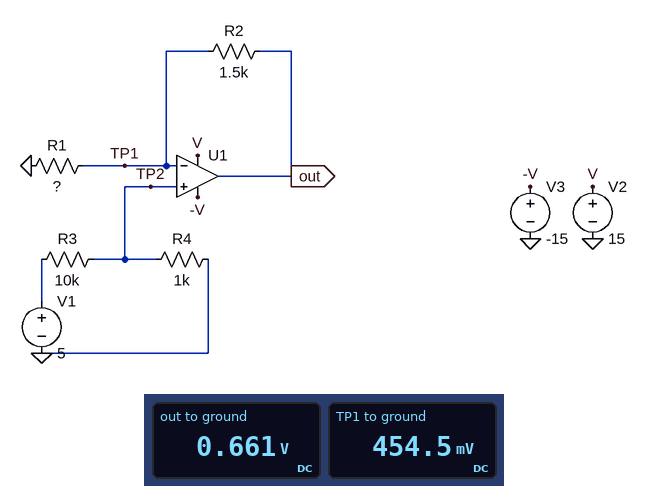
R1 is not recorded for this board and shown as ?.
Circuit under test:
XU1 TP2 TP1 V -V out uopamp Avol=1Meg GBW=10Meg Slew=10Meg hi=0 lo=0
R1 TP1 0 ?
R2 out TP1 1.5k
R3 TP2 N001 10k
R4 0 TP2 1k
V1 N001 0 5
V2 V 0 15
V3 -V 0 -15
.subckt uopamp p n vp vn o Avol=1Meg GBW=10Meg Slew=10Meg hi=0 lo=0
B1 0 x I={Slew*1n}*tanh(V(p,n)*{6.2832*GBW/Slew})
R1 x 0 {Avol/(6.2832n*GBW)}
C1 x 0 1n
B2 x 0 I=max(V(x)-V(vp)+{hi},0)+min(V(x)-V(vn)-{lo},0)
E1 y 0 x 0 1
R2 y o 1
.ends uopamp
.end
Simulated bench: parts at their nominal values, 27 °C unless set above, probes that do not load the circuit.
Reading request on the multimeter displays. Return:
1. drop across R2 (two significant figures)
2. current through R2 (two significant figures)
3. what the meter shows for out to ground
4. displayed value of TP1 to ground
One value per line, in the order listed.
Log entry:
210 mV
140 µA
0.661 V
454.5 mV
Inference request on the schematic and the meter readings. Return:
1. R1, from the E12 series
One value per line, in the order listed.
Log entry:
3.3 kΩ
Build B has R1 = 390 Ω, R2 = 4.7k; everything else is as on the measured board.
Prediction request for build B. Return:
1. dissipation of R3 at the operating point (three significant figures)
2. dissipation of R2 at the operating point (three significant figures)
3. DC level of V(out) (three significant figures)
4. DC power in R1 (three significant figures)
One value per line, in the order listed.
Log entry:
2.07 mW
6.38 mW
5.93 V
530 µW
